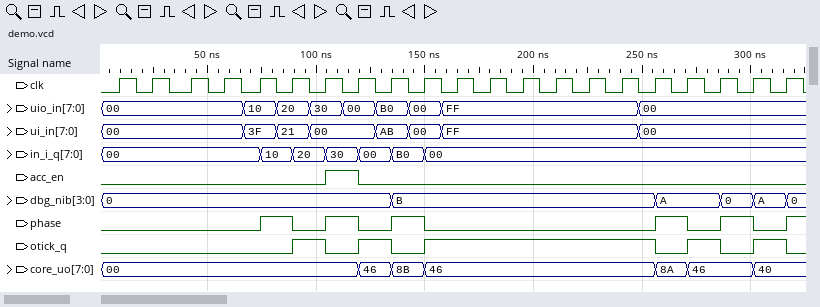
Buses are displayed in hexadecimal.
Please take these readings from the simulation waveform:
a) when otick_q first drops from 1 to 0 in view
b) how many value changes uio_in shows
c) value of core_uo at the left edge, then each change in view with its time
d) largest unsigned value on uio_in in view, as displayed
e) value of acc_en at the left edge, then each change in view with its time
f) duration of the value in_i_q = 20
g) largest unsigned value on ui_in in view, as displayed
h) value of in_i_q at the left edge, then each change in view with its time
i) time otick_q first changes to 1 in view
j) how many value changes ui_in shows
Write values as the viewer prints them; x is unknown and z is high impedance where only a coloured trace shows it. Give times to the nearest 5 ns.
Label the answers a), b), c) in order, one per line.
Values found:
a) 105 ns
b) 8
c) 00, 46 at 120 ns, 8B at 135 ns, 46 at 150 ns, 8A at 255 ns, 46 at 270 ns, 40 at 300 ns
d) FF
e) 0, 1 at 105 ns, 0 at 120 ns
f) 15 ns
g) FF
h) 00, 10 at 75 ns, 20 at 90 ns, 30 at 105 ns, 00 at 120 ns, B0 at 135 ns, 00 at 150 ns
i) 90 ns
j) 7
